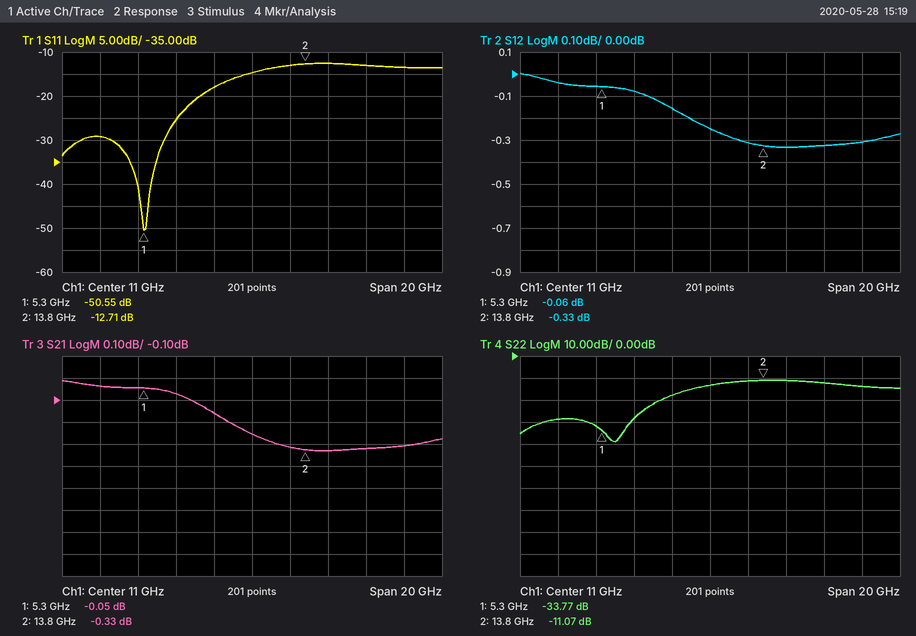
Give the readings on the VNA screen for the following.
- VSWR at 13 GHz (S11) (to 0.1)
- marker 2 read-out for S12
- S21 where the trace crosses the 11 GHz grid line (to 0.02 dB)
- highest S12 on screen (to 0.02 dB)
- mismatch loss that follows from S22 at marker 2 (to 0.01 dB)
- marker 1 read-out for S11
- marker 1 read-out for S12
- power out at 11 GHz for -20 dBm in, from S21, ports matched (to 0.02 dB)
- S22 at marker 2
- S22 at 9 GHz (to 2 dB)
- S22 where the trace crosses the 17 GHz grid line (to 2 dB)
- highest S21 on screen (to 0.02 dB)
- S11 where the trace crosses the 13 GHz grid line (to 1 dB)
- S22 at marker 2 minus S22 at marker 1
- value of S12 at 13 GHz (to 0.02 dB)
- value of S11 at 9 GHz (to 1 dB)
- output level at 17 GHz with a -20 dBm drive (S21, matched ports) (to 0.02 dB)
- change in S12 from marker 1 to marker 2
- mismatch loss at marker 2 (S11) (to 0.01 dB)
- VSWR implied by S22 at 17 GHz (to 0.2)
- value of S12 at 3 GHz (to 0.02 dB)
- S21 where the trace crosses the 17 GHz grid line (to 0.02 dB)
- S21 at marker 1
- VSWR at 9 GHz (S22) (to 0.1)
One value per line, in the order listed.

1.6
-0.33 dB
-0.26 dB
0.00 dB
0.35 dB
-50.55 dB
-0.06 dB
-20.26 dBm
-11.07 dB
-18 dB
-12 dB
-0.02 dB
-13 dB
22.70 dB
-0.32 dB
-18 dB
-20.32 dBm
-0.27 dB
0.24 dB
1.6
-0.04 dB
-0.32 dB
-0.05 dB
1.3
